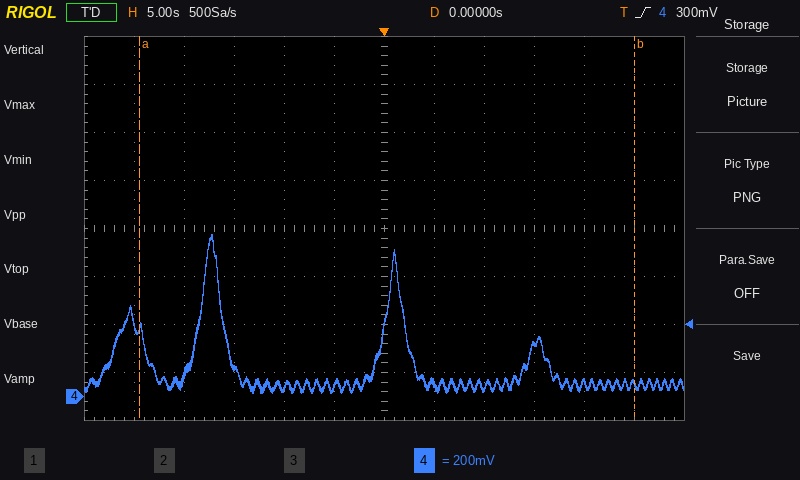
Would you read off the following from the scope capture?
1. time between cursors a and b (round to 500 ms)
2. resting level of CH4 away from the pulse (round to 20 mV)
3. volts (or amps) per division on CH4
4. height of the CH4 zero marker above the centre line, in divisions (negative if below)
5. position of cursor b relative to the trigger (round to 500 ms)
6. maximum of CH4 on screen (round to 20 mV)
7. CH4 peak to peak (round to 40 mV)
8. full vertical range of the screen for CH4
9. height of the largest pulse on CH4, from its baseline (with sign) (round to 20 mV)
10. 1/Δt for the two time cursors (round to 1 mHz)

49.5 s
60 mV
200 mV
-3.5 div
+25.0 s
680 mV
680 mV
1.6 V
+620 mV
20 mHz
